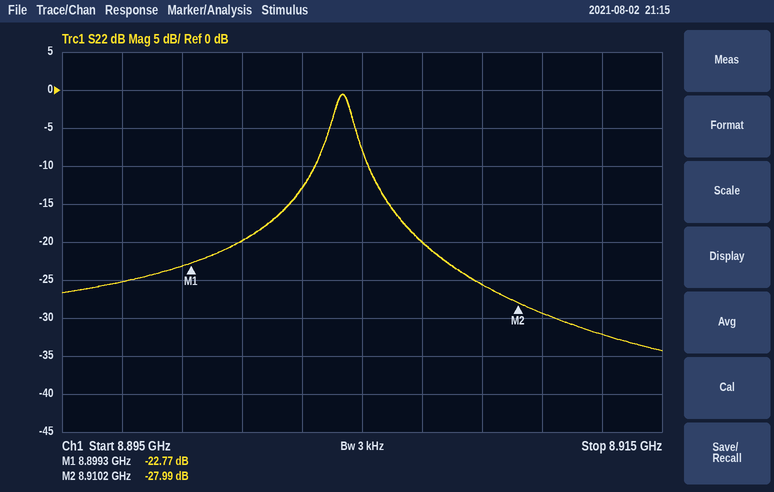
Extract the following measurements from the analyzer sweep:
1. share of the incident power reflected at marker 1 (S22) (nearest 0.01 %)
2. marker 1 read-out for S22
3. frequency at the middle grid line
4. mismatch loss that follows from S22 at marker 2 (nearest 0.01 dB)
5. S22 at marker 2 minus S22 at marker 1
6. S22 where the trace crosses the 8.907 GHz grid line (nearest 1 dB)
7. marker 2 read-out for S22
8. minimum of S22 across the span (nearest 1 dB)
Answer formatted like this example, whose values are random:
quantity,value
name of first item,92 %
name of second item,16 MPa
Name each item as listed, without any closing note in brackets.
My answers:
quantity,value
share of the incident power reflected at marker 1 (S22),0.53 %
marker 1 read-out for S22,-22.77 dB
frequency at the middle grid line,8.905 GHz
mismatch loss that follows from S22 at marker 2,0.01 dB
S22 at marker 2 minus S22 at marker 1,-5.22 dB
S22 where the trace crosses the 8.907 GHz grid line,-20 dB
marker 2 read-out for S22,-27.99 dB
minimum of S22 across the span,-34 dB
